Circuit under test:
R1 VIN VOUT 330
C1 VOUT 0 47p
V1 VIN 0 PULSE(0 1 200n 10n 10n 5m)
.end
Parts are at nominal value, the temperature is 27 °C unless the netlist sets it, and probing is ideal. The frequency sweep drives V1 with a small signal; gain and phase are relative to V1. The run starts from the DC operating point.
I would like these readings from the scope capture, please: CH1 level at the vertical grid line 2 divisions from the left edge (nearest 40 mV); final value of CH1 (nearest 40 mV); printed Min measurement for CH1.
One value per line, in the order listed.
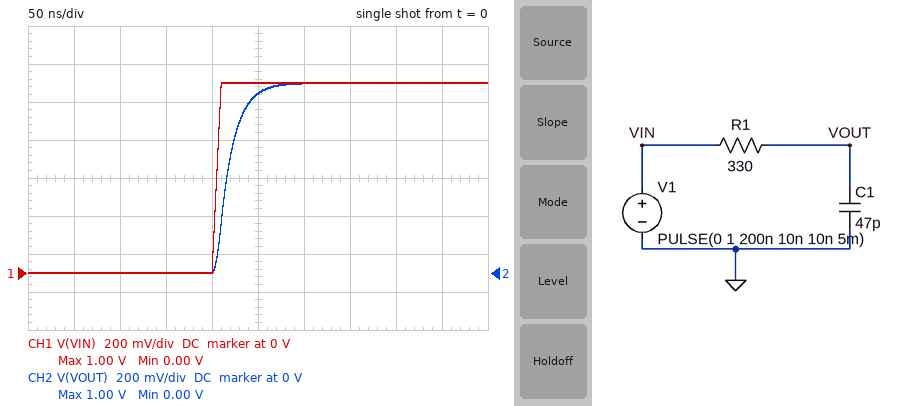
0 V
1.00 V
0.00 V
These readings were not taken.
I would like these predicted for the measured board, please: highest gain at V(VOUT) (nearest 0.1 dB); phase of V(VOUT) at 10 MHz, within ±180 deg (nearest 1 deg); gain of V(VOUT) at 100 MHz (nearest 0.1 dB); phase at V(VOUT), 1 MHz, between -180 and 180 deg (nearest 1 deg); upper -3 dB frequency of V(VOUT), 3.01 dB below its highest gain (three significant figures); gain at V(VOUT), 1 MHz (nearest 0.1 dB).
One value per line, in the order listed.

0 dB
-44 deg
-19.8 dB
-6 deg
10.3 MHz
0 dB
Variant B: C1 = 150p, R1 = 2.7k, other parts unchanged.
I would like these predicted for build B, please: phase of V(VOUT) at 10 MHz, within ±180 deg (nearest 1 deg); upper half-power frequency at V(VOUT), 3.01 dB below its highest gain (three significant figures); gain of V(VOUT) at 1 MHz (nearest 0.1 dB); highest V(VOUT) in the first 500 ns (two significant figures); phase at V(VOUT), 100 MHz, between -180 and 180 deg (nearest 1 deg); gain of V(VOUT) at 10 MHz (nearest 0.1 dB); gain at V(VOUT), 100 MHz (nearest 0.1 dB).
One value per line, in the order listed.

-88 deg
393 kHz
-8.7 dB
520 mV
-90 deg
-28.1 dB
-48.1 dB
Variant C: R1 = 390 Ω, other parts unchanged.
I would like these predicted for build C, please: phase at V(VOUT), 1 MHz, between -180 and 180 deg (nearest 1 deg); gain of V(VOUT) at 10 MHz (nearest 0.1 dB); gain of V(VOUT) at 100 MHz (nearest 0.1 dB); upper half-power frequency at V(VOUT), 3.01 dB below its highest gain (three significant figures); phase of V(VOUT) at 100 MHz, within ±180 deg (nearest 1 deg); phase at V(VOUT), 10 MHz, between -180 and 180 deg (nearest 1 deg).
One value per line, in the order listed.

-7 deg
-3.7 dB
-21.3 dB
8.68 MHz
-85 deg
-49 deg
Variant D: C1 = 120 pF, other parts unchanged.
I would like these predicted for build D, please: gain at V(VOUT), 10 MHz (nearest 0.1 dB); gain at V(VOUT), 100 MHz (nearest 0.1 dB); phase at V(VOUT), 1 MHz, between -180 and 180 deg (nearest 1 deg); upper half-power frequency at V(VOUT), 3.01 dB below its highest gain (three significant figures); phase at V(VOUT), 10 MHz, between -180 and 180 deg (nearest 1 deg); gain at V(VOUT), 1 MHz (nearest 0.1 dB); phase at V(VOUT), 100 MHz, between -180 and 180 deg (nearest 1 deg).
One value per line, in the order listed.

-8.6 dB
-27.9 dB
-14 deg
4.02 MHz
-68 deg
-0.3 dB
-88 deg
